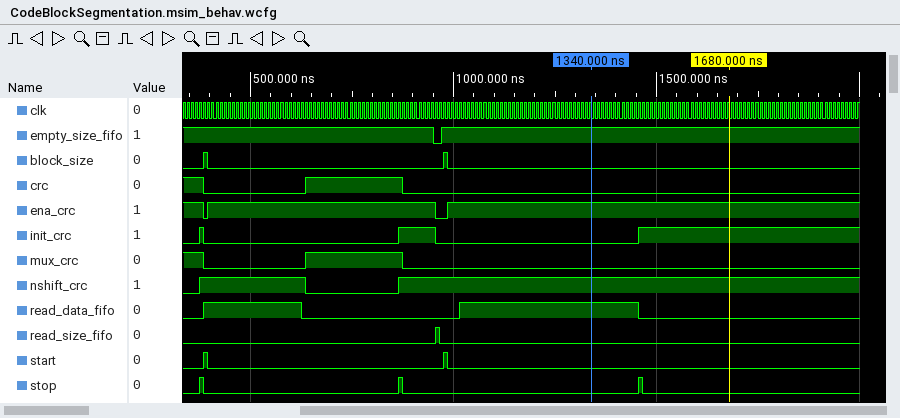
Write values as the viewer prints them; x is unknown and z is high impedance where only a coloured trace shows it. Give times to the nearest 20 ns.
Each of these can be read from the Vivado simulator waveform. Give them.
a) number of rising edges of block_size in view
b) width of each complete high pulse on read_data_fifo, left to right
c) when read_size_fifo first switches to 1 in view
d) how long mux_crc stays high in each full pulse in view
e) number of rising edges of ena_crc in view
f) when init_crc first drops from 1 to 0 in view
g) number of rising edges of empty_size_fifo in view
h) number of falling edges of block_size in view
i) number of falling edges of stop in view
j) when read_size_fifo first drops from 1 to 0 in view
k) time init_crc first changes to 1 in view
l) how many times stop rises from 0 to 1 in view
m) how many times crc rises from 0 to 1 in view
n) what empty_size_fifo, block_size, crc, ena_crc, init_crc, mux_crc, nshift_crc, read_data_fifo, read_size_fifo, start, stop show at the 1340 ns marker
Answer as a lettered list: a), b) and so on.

a) 2
b) 240 ns, 440 ns
c) 960 ns
d) 240 ns
e) 2
f) 380 ns
g) 1
h) 2
i) 3
j) 960 ns
k) 380 ns
l) 3
m) 1
n) empty_size_fifo=1, block_size=0, crc=0, ena_crc=1, init_crc=0, mux_crc=0, nshift_crc=1, read_data_fifo=1, read_size_fifo=0, start=0, stop=0
